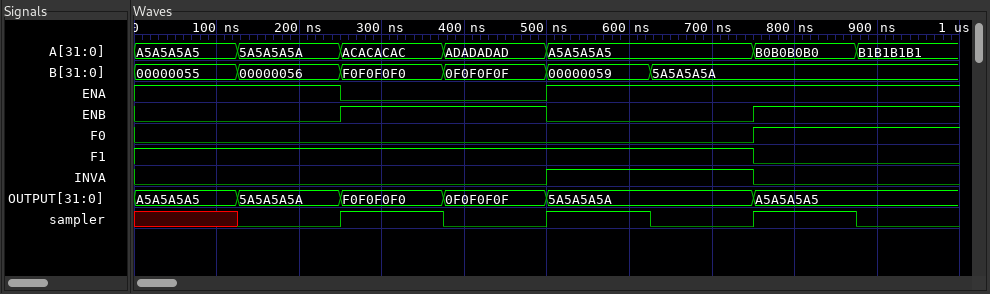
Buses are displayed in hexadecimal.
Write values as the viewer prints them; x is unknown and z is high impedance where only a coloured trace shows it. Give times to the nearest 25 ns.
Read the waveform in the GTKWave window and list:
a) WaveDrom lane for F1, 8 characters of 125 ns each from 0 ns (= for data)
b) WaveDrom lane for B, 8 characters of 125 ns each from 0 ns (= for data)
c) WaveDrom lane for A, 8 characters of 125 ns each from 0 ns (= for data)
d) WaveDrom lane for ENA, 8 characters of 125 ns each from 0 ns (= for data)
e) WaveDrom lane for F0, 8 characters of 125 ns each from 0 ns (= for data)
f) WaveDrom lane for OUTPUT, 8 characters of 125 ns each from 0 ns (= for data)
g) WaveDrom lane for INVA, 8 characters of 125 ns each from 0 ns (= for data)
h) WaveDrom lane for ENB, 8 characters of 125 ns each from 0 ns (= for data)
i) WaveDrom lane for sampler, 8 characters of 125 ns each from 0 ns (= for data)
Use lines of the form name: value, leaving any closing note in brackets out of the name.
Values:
WaveDrom lane for F1, 8 characters of 125 ns each from 0 ns: {name: 'F1', wave: '1.....0.'}
WaveDrom lane for B, 8 characters of 125 ns each from 0 ns: {name: 'B', wave: '======..', data: '00000055 00000056 F0F0F0F0 0F0F0F0F 00000059 5A5A5A5A'}
WaveDrom lane for A, 8 characters of 125 ns each from 0 ns: {name: 'A', wave: '=====.==', data: 'A5A5A5A5 5A5A5A5A ACACACAC ADADADAD A5A5A5A5 B0B0B0B0 B1B1B1B1'}
WaveDrom lane for ENA, 8 characters of 125 ns each from 0 ns: {name: 'ENA', wave: '1.0.1...'}
WaveDrom lane for F0, 8 characters of 125 ns each from 0 ns: {name: 'F0', wave: '0.....1.'}
WaveDrom lane for OUTPUT, 8 characters of 125 ns each from 0 ns: {name: 'OUTPUT', wave: '=====.=.', data: 'A5A5A5A5 5A5A5A5A F0F0F0F0 0F0F0F0F 5A5A5A5A A5A5A5A5'}
WaveDrom lane for INVA, 8 characters of 125 ns each from 0 ns: {name: 'INVA', wave: '0...1.0.'}
WaveDrom lane for ENB, 8 characters of 125 ns each from 0 ns: {name: 'ENB', wave: '0.1.0.1.'}
WaveDrom lane for sampler, 8 characters of 125 ns each from 0 ns: {name: 'sampler', wave: 'x0101010'}
